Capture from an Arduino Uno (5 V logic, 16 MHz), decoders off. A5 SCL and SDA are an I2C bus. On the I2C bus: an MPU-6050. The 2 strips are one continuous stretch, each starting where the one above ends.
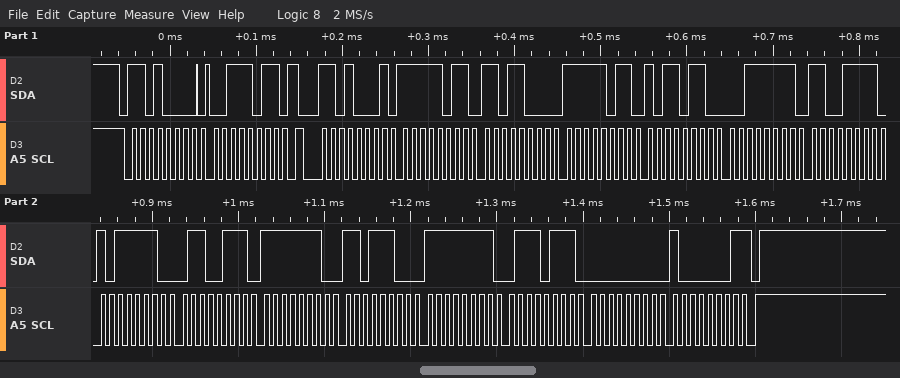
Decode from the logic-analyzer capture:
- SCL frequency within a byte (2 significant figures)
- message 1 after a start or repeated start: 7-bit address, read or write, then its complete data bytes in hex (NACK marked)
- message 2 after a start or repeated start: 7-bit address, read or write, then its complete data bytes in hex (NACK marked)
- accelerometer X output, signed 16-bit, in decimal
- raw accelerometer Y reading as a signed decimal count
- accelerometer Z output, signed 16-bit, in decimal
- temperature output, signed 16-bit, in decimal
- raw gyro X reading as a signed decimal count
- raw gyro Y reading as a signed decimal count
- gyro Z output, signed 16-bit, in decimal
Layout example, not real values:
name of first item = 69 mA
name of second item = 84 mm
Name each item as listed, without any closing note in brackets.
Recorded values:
SCL frequency within a byte = 100 kHz
message 1 after a start or repeated start: 7-bit address, read or write, then its complete data bytes in hex = 0x68 write: 3B
message 2 after a start or repeated start: 7-bit address, read or write, then its complete data bytes in hex = 0x68 read: FB D8 FB B6 3F CF BE 67 FE DC FF 77 00 81 NACK
accelerometer X output, signed 16-bit, in decimal = -1064
raw accelerometer Y reading as a signed decimal count = -1098
accelerometer Z output, signed 16-bit, in decimal = 16335
temperature output, signed 16-bit, in decimal = -16793
raw gyro X reading as a signed decimal count = -292
raw gyro Y reading as a signed decimal count = -137
gyro Z output, signed 16-bit, in decimal = 129
